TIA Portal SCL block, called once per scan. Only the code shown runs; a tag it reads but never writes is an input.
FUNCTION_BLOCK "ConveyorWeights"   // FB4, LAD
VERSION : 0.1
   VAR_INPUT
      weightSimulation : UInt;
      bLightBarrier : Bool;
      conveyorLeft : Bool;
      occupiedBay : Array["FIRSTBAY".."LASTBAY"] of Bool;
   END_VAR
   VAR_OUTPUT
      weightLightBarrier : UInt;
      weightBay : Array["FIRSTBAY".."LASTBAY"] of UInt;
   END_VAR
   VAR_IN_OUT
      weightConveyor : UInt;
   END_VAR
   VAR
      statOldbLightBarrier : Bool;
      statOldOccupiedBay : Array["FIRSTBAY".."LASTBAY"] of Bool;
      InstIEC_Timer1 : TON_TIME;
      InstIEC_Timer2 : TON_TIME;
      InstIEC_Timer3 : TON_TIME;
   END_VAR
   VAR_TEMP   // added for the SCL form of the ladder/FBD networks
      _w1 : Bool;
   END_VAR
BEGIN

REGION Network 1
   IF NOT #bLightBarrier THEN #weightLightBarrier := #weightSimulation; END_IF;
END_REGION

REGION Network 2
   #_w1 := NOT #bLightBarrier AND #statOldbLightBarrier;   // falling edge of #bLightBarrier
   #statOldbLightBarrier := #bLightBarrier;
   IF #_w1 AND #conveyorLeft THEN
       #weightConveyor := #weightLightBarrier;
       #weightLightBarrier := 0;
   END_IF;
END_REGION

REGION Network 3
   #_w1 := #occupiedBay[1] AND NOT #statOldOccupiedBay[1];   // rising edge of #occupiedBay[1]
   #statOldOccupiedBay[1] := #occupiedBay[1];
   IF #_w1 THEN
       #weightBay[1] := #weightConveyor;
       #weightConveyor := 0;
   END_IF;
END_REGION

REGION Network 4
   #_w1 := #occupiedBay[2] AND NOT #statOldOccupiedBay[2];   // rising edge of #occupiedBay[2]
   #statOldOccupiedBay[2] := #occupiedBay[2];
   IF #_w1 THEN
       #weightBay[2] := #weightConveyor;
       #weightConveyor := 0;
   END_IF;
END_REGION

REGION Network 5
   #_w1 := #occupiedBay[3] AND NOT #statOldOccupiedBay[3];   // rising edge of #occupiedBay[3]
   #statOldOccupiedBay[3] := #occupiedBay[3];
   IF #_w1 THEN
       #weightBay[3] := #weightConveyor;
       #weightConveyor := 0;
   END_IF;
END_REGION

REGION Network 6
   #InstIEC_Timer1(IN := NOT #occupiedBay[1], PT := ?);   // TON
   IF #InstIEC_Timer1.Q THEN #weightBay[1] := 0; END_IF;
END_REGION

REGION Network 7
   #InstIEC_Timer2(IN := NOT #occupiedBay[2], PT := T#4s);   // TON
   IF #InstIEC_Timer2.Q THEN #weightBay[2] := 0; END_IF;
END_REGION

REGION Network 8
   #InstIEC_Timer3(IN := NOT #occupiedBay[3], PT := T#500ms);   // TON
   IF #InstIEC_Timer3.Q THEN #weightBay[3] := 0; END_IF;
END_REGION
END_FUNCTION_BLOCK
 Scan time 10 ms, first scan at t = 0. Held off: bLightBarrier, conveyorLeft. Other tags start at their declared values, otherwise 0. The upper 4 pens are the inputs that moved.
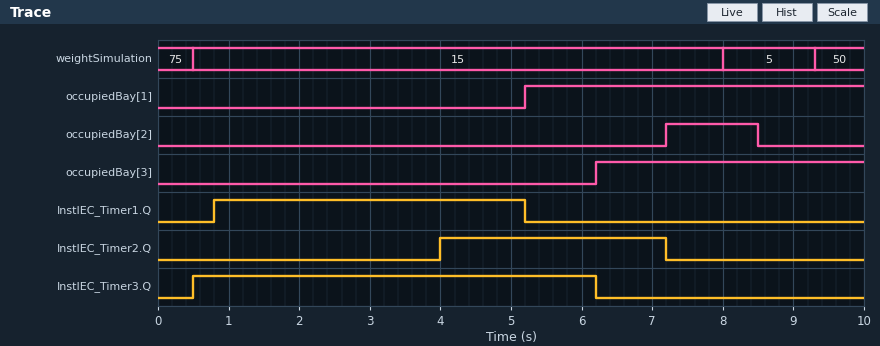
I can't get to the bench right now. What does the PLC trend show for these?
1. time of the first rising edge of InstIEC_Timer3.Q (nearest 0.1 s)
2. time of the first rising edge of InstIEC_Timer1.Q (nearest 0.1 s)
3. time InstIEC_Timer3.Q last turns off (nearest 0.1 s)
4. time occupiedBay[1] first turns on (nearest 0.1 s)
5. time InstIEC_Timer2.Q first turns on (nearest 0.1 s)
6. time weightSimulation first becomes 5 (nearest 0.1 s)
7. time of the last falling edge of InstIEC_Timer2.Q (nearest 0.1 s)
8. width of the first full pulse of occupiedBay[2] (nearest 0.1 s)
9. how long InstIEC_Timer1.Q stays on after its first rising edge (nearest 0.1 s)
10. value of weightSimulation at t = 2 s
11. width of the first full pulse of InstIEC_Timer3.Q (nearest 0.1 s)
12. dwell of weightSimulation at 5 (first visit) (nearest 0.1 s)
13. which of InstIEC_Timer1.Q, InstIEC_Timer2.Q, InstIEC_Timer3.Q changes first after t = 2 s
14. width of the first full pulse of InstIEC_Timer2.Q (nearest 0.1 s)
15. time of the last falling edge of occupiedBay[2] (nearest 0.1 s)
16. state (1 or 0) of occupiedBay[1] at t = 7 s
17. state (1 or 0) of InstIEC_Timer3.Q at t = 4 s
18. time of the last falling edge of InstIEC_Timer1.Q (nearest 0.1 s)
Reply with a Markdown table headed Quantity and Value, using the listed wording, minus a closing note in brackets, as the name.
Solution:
| Quantity | Value |
|---|---|
| time of the first rising edge of InstIEC_Timer3.Q | 0.5 s |
| time of the first rising edge of InstIEC_Timer1.Q | 0.8 s |
| time InstIEC_Timer3.Q last turns off | 6.2 s |
| time occupiedBay[1] first turns on | 5.2 s |
| time InstIEC_Timer2.Q first turns on | 4.0 s |
| time weightSimulation first becomes 5 | 8.0 s |
| time of the last falling edge of InstIEC_Timer2.Q | 7.2 s |
| width of the first full pulse of occupiedBay[2] | 1.3 s |
| how long InstIEC_Timer1.Q stays on after its first rising edge | 4.4 s |
| value of weightSimulation at t = 2 s | 15 |
| width of the first full pulse of InstIEC_Timer3.Q | 5.7 s |
| dwell of weightSimulation at 5 (first visit) | 1.3 s |
| which of InstIEC_Timer1.Q, InstIEC_Timer2.Q, InstIEC_Timer3.Q changes first after t = 2 s | InstIEC_Timer2.Q |
| width of the first full pulse of InstIEC_Timer2.Q | 3.2 s |
| time of the last falling edge of occupiedBay[2] | 8.5 s |
| state (1 or 0) of occupiedBay[1] at t = 7 s | 1 |
| state (1 or 0) of InstIEC_Timer3.Q at t = 4 s | 1 |
| time of the last falling edge of InstIEC_Timer1.Q | 5.2 s |
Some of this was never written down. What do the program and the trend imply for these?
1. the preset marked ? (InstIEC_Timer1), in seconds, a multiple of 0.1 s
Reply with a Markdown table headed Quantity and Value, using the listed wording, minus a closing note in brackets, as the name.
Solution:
| Quantity | Value |
|---|---|
| the preset marked ? (InstIEC_Timer1), in seconds, a multiple of 0.1 s | 0.8 s |
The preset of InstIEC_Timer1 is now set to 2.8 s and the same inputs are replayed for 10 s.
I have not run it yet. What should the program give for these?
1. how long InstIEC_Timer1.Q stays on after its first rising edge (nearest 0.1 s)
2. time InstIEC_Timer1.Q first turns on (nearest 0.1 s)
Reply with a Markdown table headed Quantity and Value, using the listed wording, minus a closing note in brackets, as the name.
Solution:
| Quantity | Value |
|---|---|
| how long InstIEC_Timer1.Q stays on after its first rising edge | 2.4 s |
| time InstIEC_Timer1.Q first turns on | 2.8 s |
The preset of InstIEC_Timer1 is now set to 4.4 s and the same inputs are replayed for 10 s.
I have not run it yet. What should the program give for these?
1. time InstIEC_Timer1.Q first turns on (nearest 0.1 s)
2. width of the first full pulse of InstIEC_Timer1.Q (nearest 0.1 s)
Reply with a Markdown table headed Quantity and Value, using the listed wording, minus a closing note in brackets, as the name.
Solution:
| Quantity | Value |
|---|---|
| time InstIEC_Timer1.Q first turns on | 4.4 s |
| width of the first full pulse of InstIEC_Timer1.Q | 0.8 s |
